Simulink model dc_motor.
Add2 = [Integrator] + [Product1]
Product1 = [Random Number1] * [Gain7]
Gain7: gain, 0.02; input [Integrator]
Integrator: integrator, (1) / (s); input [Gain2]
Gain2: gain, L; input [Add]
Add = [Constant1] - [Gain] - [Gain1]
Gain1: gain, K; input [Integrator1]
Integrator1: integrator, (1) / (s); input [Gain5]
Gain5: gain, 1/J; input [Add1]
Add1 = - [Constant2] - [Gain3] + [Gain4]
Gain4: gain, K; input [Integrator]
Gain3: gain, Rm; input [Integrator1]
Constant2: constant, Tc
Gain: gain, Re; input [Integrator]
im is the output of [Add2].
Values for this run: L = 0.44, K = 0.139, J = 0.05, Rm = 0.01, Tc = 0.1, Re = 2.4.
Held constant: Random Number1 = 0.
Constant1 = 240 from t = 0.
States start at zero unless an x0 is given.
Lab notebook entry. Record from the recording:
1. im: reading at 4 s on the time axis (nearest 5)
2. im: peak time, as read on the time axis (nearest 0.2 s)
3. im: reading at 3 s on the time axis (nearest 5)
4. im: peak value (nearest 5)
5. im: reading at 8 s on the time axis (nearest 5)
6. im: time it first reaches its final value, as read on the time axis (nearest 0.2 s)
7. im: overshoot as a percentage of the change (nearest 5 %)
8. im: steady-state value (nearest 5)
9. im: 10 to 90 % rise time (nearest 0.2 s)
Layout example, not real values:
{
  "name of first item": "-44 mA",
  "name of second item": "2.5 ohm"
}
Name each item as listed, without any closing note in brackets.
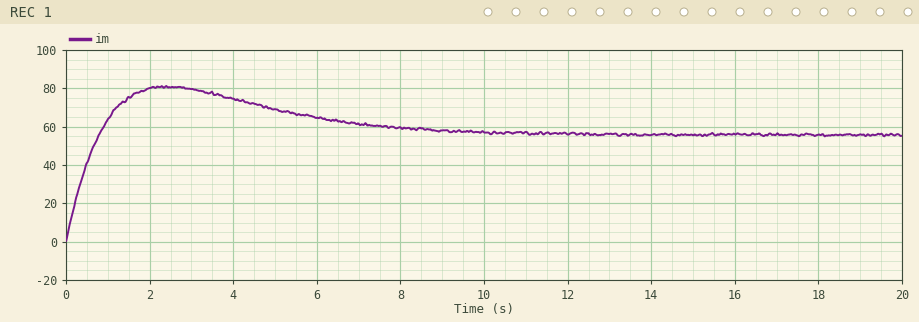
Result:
{
  "im: reading at 4 s on the time axis": "75",
  "im: peak time, as read on the time axis": "2.4 s",
  "im: reading at 3 s on the time axis": "80",
  "im: peak value": "80",
  "im: reading at 8 s on the time axis": "60",
  "im: time it first reaches its final value, as read on the time axis": "0.8 s",
  "im: overshoot as a percentage of the change": "45 %",
  "im: steady-state value": "55",
  "im: 10 to 90 % rise time": "0.6 s"
}
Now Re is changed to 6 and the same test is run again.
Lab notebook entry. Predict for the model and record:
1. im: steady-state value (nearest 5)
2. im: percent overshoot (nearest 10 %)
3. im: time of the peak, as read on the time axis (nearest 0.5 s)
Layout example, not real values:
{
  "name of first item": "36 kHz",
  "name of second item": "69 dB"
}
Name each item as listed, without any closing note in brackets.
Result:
{
  "im: steady-state value": "30",
  "im: percent overshoot": "20 %",
  "im: time of the peak, as read on the time axis": "1.5 s"
}
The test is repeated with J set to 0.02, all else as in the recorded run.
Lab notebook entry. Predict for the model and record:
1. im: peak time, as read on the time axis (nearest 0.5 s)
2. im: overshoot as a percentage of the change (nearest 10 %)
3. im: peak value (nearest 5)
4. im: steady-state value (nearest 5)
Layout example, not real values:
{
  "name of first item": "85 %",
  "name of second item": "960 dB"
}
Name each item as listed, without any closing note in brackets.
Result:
{
  "im: peak time, as read on the time axis": "2.0 s",
  "im: overshoot as a percentage of the change": "30 %",
  "im: peak value": "70",
  "im: steady-state value": "55"
}
